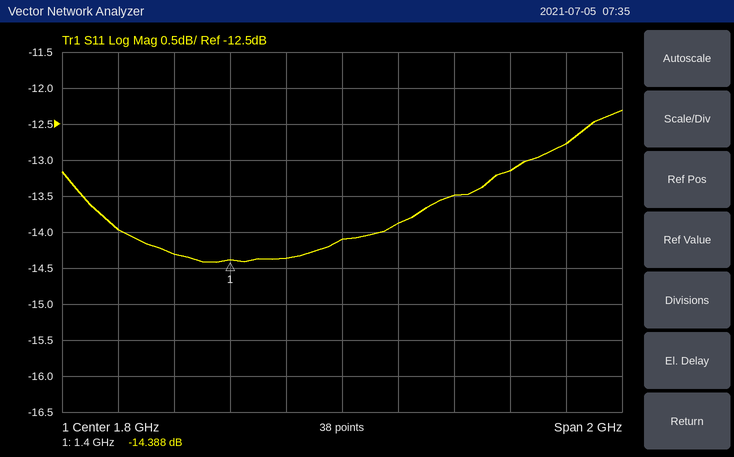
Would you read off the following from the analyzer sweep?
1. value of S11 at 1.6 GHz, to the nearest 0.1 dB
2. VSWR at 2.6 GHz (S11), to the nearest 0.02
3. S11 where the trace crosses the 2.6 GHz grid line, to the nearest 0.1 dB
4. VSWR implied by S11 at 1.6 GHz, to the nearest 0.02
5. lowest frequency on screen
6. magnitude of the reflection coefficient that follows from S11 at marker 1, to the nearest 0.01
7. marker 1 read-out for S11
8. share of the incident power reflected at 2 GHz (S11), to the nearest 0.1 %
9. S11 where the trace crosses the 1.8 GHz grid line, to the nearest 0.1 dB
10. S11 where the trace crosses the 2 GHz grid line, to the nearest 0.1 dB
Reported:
-14.4 dB
1.60
-12.8 dB
1.48
800 MHz
0.19
-14.388 dB
4.1 %
-14.1 dB
-13.9 dB
